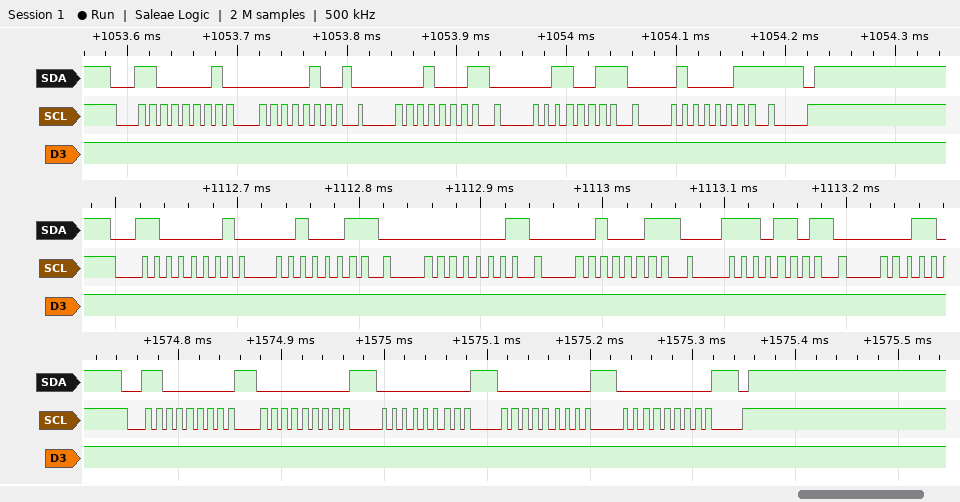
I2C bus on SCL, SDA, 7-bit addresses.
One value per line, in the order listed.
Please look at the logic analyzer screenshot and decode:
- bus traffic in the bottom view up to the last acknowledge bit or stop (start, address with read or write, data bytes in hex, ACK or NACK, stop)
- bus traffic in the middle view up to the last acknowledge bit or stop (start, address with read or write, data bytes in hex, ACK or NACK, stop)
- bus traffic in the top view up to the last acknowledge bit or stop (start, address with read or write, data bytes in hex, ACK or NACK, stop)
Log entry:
start, address 60 write ACK, 00 ACK, 00 ACK, 00 ACK, 00 ACK, stop
start, address 60 read ACK, 23 ACK, 01 ACK, 23 ACK, ED ACK
start, address 60 read ACK, 04 ACK, 11 ACK, 33 ACK, 43 NACK, stop
